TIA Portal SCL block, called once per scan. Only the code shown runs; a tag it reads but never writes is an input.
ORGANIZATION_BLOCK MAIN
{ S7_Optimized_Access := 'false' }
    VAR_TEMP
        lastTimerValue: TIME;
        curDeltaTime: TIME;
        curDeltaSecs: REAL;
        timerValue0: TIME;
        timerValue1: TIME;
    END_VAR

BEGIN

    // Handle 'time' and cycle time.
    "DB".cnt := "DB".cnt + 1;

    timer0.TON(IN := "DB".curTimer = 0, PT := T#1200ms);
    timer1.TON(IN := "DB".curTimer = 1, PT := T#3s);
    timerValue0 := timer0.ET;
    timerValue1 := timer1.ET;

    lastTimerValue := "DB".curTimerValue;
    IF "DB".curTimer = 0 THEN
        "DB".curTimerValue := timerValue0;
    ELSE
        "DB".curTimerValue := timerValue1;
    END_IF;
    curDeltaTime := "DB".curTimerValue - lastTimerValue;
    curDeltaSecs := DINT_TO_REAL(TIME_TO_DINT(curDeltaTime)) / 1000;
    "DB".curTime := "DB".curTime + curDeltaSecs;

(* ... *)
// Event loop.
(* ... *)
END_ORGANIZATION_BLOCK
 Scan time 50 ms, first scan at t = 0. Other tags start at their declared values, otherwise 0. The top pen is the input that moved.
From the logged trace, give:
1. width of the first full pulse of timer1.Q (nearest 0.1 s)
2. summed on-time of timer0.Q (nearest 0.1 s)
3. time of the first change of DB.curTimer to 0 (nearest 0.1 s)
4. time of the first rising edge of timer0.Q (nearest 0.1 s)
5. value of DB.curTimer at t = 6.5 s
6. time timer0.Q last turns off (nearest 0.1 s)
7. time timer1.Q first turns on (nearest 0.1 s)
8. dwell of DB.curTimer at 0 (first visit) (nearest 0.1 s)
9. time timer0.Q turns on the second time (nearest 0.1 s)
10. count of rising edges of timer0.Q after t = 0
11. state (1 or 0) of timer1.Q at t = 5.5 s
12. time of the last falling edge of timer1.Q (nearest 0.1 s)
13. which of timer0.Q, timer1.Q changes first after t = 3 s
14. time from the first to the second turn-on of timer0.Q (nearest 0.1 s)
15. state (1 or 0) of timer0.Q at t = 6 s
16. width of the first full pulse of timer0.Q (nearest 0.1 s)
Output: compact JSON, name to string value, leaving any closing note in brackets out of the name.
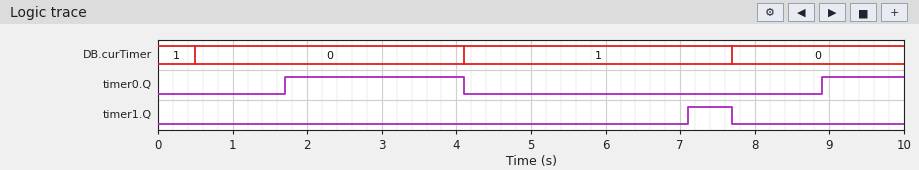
{"width of the first full pulse of timer1.Q": "0.6 s", "summed on-time of timer0.Q": "3.5 s", "time of the first change of DB.curTimer to 0": "0.5 s", "time of the first rising edge of timer0.Q": "1.7 s", "value of DB.curTimer at t = 6.5 s": "1", "time timer0.Q last turns off": "4.1 s", "time timer1.Q first turns on": "7.1 s", "dwell of DB.curTimer at 0 (first visit)": "3.6 s", "time timer0.Q turns on the second time": "8.9 s", "count of rising edges of timer0.Q after t = 0": "2", "state (1 or 0) of timer1.Q at t = 5.5 s": "0", "time of the last falling edge of timer1.Q": "7.7 s", "which of timer0.Q, timer1.Q changes first after t = 3 s": "timer0.Q", "time from the first to the second turn-on of timer0.Q": "7.2 s", "state (1 or 0) of timer0.Q at t = 6 s": "0", "width of the first full pulse of timer0.Q": "2.4 s"}
